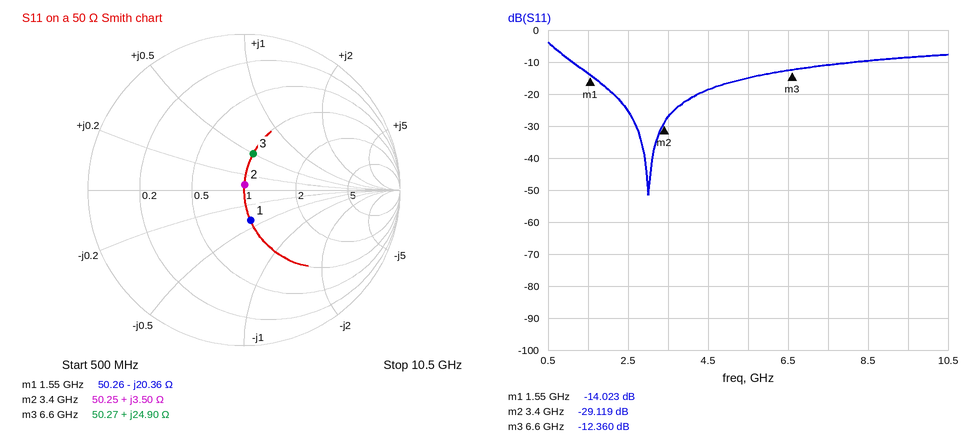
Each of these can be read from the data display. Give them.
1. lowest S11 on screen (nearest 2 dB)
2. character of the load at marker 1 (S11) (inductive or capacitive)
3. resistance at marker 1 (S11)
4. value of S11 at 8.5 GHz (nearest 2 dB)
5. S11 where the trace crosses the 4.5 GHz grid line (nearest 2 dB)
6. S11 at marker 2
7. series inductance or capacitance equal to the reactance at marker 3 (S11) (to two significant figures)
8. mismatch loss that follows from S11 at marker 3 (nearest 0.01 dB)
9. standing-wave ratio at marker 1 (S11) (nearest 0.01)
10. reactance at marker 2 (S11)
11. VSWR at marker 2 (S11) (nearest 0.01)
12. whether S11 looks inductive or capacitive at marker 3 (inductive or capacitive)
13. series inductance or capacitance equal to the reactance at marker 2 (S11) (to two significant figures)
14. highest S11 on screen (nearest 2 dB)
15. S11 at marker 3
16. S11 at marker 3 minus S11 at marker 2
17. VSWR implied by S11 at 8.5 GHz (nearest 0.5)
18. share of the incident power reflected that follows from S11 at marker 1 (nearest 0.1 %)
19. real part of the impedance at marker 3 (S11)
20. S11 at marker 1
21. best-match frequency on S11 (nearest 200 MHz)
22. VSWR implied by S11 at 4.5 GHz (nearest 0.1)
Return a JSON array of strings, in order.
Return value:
["-52 dB", "capacitive", "50.26 Ω", "-10 dB", "-18 dB", "-29.119 dB", "600 pH", "0.26 dB", "1.50", "+3.50 Ω", "1.07", "inductive", "160 pH", "-4 dB", "-12.360 dB", "16.759 dB", "2.0", "4.0 %", "50.27 Ω", "-14.023 dB", "3.0 GHz", "1.3"]
